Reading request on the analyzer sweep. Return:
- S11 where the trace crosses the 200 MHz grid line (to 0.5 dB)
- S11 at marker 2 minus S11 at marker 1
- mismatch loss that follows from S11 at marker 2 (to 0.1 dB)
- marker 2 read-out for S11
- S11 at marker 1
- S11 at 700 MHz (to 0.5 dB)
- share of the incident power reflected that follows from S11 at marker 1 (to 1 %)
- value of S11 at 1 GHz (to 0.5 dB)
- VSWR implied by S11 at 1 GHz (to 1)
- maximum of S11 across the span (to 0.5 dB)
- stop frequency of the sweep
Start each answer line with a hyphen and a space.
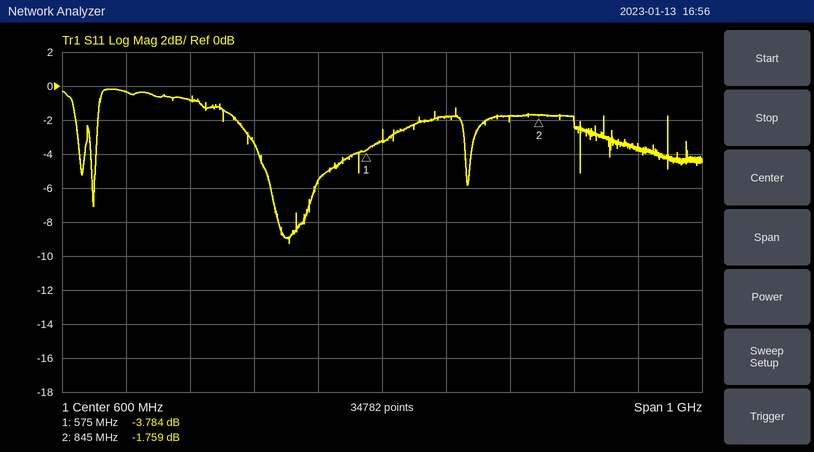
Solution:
- -0.5 dB
- 2.025 dB
- 4.8 dB
- -1.759 dB
- -3.784 dB
- -2.0 dB
- 42 %
- -3.5 dB
- 5
- 0.0 dB
- 1.1 GHz
